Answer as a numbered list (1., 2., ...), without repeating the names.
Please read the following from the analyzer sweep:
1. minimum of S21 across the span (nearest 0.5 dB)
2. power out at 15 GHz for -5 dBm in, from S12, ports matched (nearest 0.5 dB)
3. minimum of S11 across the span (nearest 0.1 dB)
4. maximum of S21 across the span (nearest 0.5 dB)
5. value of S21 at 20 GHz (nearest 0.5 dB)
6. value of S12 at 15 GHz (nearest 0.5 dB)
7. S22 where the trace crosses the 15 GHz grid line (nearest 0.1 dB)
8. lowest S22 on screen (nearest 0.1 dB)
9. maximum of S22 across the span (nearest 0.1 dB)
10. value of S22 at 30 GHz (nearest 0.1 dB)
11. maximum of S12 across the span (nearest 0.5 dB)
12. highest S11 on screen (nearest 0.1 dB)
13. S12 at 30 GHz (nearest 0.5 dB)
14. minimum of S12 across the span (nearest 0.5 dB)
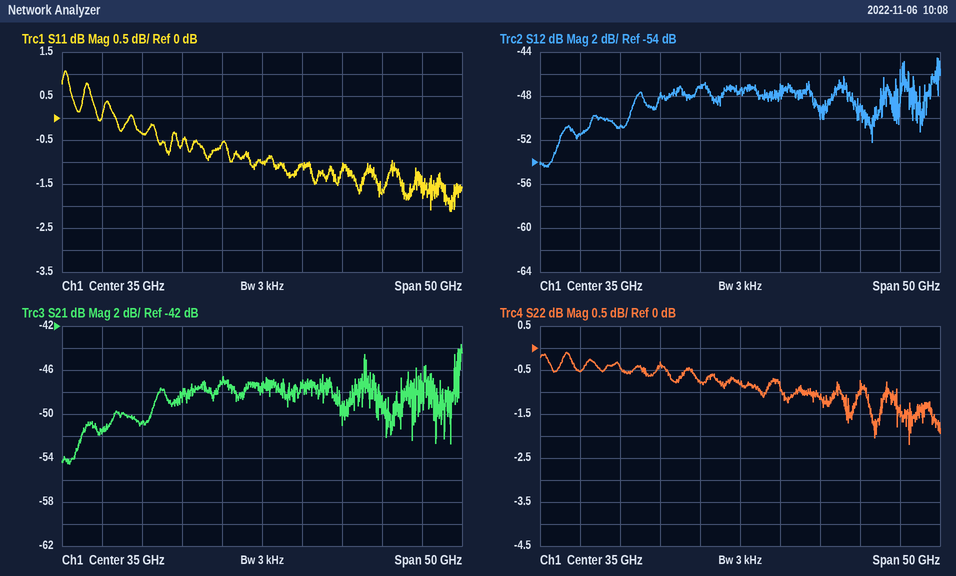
1. -54.5 dB
2. -56.5 dBm
3. -2.1 dB
4. -43.5 dB
5. -51.0 dB
6. -51.5 dB
7. -0.5 dB
8. -2.2 dB
9. -0.1 dB
10. -0.8 dB
11. -44.5 dB
12. 1.1 dB
13. -47.0 dB
14. -54.5 dB
